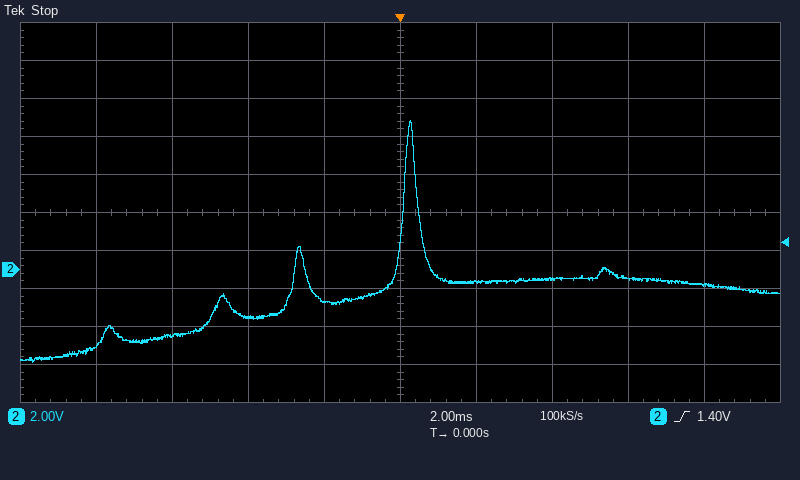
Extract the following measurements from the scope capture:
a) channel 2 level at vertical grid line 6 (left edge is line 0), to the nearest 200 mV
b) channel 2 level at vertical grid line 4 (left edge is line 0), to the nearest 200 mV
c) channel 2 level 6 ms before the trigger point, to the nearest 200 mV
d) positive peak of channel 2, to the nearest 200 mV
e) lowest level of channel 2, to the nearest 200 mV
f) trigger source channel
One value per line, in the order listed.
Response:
-600 mV
-1.6 V
-3.4 V
7.8 V
-4.8 V
channel 2
